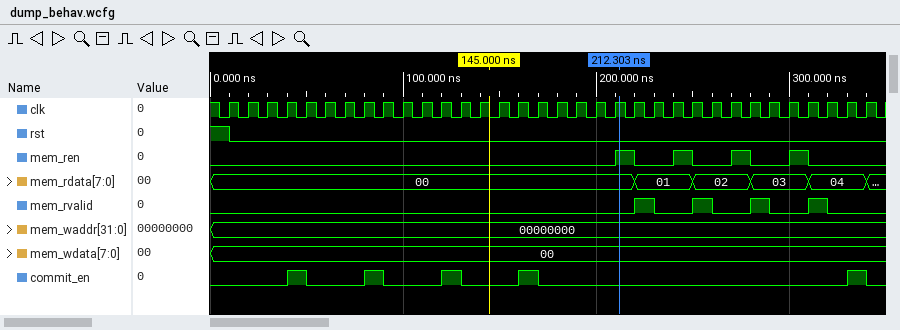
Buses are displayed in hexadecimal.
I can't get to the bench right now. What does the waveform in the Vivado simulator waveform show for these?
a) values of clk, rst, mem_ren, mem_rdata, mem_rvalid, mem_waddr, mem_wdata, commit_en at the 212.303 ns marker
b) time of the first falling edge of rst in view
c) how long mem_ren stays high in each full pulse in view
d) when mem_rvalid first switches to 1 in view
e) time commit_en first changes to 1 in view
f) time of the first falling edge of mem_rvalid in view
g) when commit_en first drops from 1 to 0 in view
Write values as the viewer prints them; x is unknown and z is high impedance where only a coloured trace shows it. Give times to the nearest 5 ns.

clk=1, rst=0, mem_ren=1, mem_rdata=00, mem_rvalid=0, mem_waddr=00000000, mem_wdata=00, commit_en=0
10 ns
10 ns, 10 ns, 10 ns, 10 ns
220 ns
40 ns
230 ns
50 ns
